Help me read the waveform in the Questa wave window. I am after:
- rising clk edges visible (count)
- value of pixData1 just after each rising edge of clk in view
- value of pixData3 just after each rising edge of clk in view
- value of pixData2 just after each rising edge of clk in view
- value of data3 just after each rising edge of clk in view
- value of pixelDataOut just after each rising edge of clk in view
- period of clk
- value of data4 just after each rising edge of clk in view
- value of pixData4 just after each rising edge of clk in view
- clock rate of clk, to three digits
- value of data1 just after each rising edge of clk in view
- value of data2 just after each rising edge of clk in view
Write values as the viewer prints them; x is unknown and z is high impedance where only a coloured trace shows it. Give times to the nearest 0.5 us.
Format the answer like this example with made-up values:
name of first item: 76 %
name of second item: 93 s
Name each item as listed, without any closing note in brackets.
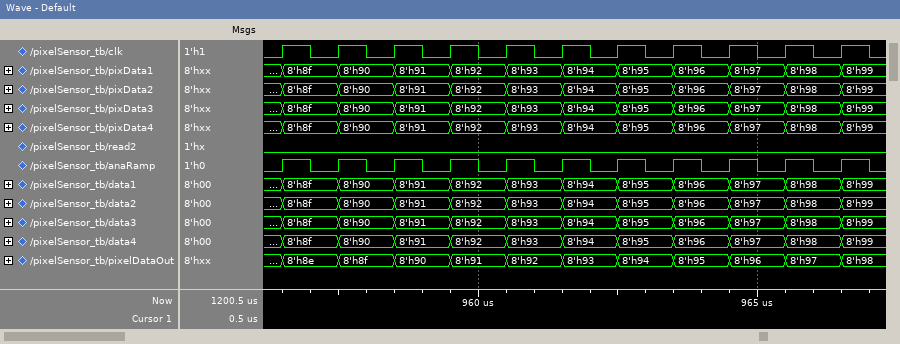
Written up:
rising clk edges visible: 11
value of pixData1 just after each rising edge of clk in view: 8'h8f, 8'h90, 8'h91, 8'h92, 8'h93, 8'h94, 8'h95, 8'h96, 8'h97, 8'h98, 8'h99
value of pixData3 just after each rising edge of clk in view: 8'h8f, 8'h90, 8'h91, 8'h92, 8'h93, 8'h94, 8'h95, 8'h96, 8'h97, 8'h98, 8'h99
value of pixData2 just after each rising edge of clk in view: 8'h8f, 8'h90, 8'h91, 8'h92, 8'h93, 8'h94, 8'h95, 8'h96, 8'h97, 8'h98, 8'h99
value of data3 just after each rising edge of clk in view: 8'h8f, 8'h90, 8'h91, 8'h92, 8'h93, 8'h94, 8'h95, 8'h96, 8'h97, 8'h98, 8'h99
value of pixelDataOut just after each rising edge of clk in view: 8'h8e, 8'h8f, 8'h90, 8'h91, 8'h92, 8'h93, 8'h94, 8'h95, 8'h96, 8'h97, 8'h98
period of clk: 1 us
value of data4 just after each rising edge of clk in view: 8'h8f, 8'h90, 8'h91, 8'h92, 8'h93, 8'h94, 8'h95, 8'h96, 8'h97, 8'h98, 8'h99
value of pixData4 just after each rising edge of clk in view: 8'h8f, 8'h90, 8'h91, 8'h92, 8'h93, 8'h94, 8'h95, 8'h96, 8'h97, 8'h98, 8'h99
clock rate of clk, to three digits: 1.00 MHz
value of data1 just after each rising edge of clk in view: 8'h8f, 8'h90, 8'h91, 8'h92, 8'h93, 8'h94, 8'h95, 8'h96, 8'h97, 8'h98, 8'h99
value of data2 just after each rising edge of clk in view: 8'h8f, 8'h90, 8'h91, 8'h92, 8'h93, 8'h94, 8'h95, 8'h96, 8'h97, 8'h98, 8'h99
